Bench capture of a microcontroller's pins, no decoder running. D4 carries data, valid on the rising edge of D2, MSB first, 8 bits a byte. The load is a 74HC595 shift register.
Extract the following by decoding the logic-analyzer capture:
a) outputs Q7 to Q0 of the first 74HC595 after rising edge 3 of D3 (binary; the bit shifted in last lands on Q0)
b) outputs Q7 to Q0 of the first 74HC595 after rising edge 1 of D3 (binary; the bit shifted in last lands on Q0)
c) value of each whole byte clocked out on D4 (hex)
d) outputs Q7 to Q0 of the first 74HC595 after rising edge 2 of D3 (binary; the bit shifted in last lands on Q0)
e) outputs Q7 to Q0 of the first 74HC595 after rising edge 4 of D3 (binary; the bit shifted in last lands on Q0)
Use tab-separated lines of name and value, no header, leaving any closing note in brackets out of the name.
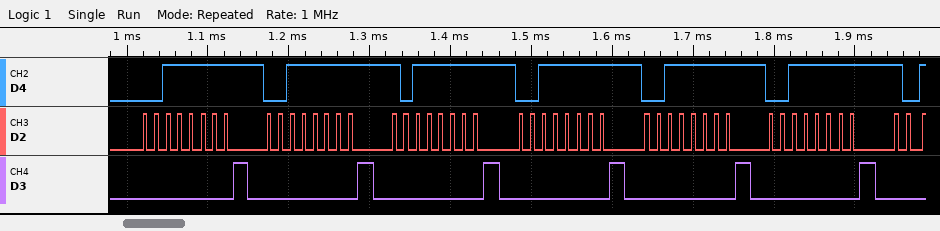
outputs Q7 to Q0 of the first 74HC595 after rising edge 3 of D3	10111111
outputs Q7 to Q0 of the first 74HC595 after rising edge 1 of D3	00111111
value of each whole byte clocked out on D4	0x3F 0x3F 0xBF 0x3F 0x3F 0x3F
outputs Q7 to Q0 of the first 74HC595 after rising edge 2 of D3	00111111
outputs Q7 to Q0 of the first 74HC595 after rising edge 4 of D3	00111111
